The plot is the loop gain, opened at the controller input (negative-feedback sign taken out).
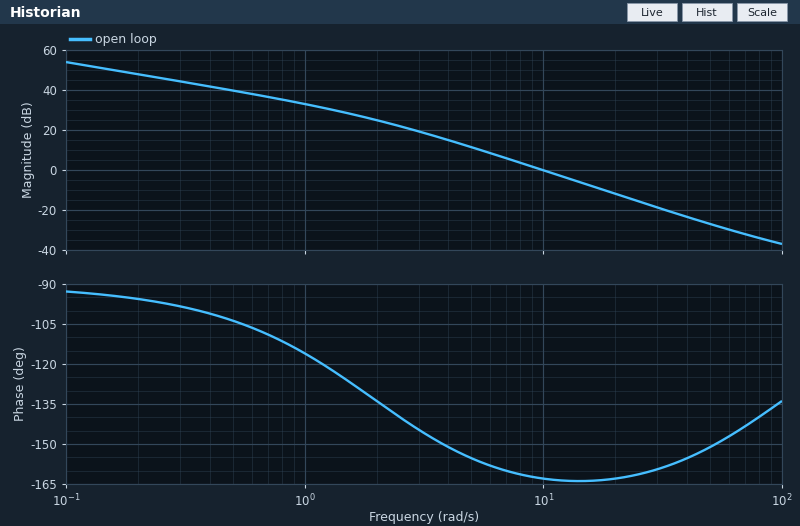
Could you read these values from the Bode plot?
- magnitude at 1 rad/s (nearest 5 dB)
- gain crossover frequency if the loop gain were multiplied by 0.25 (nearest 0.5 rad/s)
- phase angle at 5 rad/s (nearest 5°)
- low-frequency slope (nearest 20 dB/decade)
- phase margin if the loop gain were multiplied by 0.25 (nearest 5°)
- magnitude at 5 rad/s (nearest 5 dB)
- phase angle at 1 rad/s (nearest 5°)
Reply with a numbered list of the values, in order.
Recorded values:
1. 35 dB
2. 5.0 rad/s
3. -155°
4. -20 dB/decade
5. 25°
6. 10 dB
7. -115°
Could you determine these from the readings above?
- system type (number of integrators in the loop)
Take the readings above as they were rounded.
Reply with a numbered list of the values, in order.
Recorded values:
1. 1
